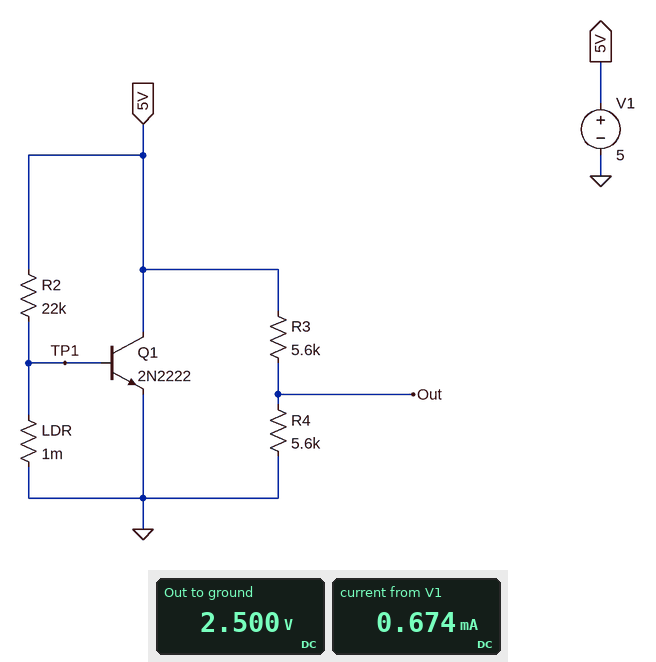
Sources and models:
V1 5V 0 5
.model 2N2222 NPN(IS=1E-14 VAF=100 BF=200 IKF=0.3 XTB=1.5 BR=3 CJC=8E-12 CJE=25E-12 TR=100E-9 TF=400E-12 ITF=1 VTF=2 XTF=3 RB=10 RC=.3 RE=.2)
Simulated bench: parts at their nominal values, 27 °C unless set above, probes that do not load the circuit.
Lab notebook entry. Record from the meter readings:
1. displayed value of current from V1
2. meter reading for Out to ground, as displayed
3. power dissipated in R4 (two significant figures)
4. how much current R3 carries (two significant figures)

0.674 mA
2.500 V
1.1 mW
450 µA
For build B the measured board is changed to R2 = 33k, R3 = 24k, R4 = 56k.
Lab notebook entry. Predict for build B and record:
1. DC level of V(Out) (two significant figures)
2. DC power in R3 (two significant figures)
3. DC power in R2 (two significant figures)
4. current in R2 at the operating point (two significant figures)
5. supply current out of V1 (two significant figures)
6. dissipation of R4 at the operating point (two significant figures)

3.5 V
94 µW
760 µW
150 µA
210 µA
220 µW
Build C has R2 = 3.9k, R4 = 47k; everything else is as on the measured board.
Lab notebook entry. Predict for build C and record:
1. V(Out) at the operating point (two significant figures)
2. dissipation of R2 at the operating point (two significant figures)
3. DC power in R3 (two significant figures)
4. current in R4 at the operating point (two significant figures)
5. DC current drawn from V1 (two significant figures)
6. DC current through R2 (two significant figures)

4.5 V
6.4 mW
51 µW
95 µA
1.4 mA
1.3 mA
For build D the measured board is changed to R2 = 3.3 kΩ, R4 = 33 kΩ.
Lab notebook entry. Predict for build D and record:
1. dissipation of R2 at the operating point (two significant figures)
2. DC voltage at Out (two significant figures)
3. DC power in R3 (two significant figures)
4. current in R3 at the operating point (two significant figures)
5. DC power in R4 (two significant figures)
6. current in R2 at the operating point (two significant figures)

7.6 mW
4.3 V
94 µW
130 µA
550 µW
1.5 mA
